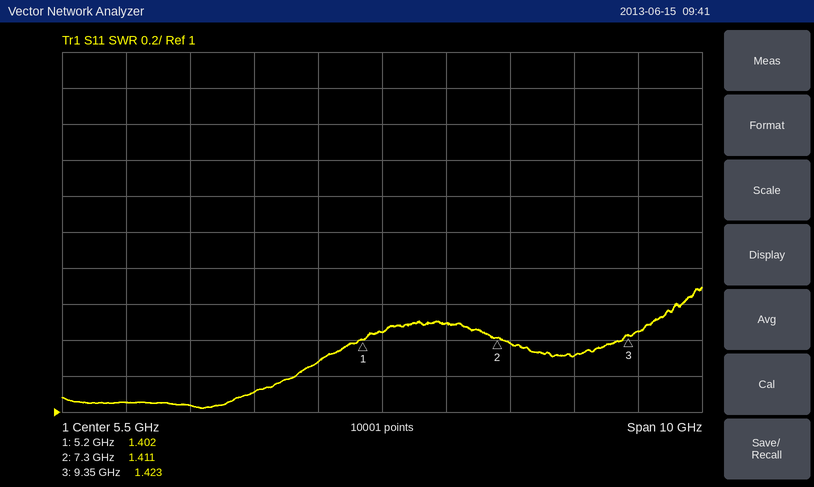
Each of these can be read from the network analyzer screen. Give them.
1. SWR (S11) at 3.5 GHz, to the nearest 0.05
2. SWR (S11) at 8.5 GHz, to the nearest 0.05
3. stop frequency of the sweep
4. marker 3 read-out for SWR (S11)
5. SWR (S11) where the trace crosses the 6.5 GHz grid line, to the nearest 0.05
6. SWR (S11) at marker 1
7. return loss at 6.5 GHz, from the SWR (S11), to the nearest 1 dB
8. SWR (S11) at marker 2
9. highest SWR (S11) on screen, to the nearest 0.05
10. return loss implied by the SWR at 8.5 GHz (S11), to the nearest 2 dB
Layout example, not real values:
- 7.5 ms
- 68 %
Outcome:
- 1.10
- 1.30
- 10.5 GHz
- 1.423
- 1.50
- 1.402
- 14 dB
- 1.411
- 1.70
- 18 dB
